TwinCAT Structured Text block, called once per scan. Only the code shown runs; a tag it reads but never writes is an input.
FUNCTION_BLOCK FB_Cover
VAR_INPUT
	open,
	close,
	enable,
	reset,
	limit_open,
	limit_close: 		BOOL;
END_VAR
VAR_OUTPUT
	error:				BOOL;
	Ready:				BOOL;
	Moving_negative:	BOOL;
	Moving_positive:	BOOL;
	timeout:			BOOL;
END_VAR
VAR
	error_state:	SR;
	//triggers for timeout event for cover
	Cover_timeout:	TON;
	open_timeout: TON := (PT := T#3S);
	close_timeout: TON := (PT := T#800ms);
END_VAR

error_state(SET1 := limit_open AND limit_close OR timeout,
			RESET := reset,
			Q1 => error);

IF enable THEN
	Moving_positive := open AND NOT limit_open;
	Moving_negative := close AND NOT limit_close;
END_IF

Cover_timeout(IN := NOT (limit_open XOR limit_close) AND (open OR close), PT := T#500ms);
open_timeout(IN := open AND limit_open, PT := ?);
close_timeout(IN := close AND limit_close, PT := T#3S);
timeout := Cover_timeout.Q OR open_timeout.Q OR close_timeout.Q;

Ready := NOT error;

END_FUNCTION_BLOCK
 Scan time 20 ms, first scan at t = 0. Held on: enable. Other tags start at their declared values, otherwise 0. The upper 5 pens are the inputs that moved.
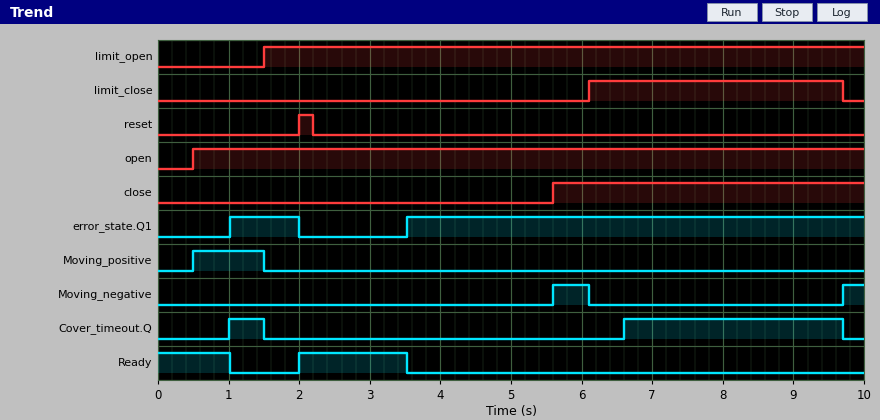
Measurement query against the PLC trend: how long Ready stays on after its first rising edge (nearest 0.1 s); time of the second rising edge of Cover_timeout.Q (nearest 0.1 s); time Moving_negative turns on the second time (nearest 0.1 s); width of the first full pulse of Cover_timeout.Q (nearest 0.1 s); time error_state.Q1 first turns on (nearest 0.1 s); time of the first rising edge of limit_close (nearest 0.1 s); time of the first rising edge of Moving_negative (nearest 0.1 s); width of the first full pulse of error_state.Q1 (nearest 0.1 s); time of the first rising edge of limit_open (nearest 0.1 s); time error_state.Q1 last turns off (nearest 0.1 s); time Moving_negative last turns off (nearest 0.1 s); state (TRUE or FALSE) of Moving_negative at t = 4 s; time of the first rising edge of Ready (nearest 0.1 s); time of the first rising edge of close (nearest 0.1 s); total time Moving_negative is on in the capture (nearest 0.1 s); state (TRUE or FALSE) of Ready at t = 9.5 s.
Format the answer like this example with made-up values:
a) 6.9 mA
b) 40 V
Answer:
a) 1.5 s
b) 6.6 s
c) 9.7 s
d) 0.5 s
e) 1.0 s
f) 6.1 s
g) 5.6 s
h) 1.0 s
i) 1.5 s
j) 2.0 s
k) 6.1 s
l) FALSE
m) 2.0 s
n) 5.6 s
o) 0.8 s
p) FALSE
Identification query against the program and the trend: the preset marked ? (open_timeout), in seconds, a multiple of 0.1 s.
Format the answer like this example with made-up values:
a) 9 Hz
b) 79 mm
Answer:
a) 2.0 s
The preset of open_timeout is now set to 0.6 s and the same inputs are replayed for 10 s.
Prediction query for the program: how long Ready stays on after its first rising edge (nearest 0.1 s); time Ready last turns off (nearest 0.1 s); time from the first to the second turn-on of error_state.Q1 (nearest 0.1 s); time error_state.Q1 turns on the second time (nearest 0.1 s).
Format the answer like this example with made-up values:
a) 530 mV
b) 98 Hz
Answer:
a) 0.1 s
b) 2.1 s
c) 1.1 s
d) 2.1 s
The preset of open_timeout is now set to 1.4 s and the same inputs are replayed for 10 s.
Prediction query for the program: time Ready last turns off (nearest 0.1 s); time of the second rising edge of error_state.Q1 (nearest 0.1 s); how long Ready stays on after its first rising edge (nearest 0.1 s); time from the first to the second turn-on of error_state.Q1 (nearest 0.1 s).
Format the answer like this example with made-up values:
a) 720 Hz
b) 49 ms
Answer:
a) 2.9 s
b) 2.9 s
c) 0.9 s
d) 1.9 s
